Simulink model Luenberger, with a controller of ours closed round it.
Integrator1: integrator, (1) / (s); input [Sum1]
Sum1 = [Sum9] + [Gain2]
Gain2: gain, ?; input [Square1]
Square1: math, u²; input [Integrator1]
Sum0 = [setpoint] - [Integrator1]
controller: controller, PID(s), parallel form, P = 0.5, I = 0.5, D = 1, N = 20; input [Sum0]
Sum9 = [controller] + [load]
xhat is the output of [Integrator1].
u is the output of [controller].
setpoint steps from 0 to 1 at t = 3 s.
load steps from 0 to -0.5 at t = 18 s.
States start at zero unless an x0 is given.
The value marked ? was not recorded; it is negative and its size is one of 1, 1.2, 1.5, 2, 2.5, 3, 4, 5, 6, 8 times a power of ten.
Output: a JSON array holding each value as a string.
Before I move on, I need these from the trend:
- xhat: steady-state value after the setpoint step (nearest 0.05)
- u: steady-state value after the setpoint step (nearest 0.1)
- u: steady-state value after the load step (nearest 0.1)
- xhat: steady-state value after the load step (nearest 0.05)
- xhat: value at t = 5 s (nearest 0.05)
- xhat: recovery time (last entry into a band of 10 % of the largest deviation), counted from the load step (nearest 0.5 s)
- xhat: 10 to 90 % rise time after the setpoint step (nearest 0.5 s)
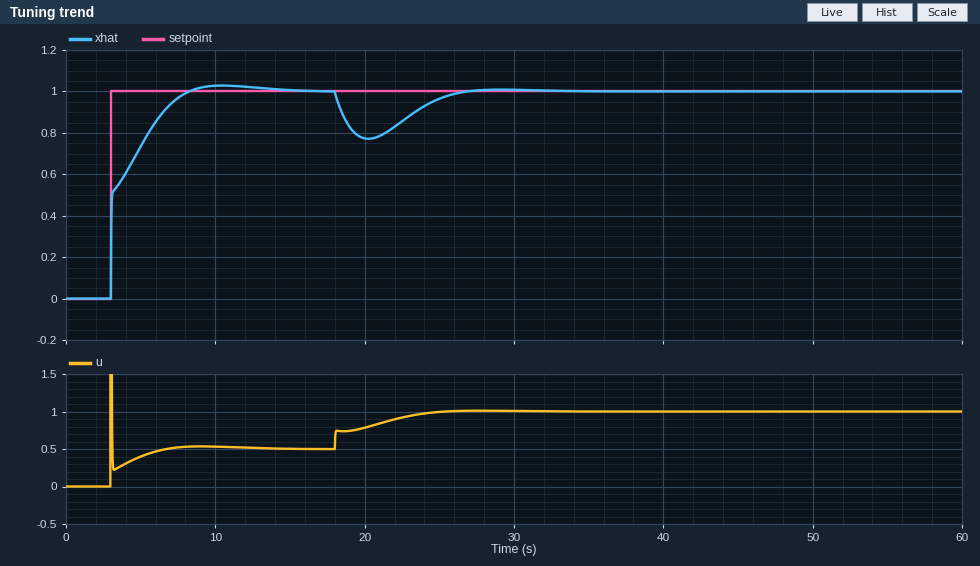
["1.00", "0.5", "1.0", "1.00", "0.75", "7.5 s", "3.5 s"]
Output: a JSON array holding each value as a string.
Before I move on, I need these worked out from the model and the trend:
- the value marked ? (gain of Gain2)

["-0.5"]
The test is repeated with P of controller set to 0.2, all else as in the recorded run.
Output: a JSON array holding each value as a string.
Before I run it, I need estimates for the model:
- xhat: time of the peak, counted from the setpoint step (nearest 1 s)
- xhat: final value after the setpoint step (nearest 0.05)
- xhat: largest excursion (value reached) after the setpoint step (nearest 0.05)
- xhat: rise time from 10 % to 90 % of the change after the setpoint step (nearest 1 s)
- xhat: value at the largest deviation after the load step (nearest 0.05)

["7 s", "1.00", "1.05", "4 s", "0.75"]
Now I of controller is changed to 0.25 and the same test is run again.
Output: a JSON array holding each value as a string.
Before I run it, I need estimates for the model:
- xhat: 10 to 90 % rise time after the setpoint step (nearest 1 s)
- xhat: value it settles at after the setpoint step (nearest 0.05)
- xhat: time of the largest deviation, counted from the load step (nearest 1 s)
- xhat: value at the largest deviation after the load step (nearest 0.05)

["6 s", "1.00", "3 s", "0.75"]
